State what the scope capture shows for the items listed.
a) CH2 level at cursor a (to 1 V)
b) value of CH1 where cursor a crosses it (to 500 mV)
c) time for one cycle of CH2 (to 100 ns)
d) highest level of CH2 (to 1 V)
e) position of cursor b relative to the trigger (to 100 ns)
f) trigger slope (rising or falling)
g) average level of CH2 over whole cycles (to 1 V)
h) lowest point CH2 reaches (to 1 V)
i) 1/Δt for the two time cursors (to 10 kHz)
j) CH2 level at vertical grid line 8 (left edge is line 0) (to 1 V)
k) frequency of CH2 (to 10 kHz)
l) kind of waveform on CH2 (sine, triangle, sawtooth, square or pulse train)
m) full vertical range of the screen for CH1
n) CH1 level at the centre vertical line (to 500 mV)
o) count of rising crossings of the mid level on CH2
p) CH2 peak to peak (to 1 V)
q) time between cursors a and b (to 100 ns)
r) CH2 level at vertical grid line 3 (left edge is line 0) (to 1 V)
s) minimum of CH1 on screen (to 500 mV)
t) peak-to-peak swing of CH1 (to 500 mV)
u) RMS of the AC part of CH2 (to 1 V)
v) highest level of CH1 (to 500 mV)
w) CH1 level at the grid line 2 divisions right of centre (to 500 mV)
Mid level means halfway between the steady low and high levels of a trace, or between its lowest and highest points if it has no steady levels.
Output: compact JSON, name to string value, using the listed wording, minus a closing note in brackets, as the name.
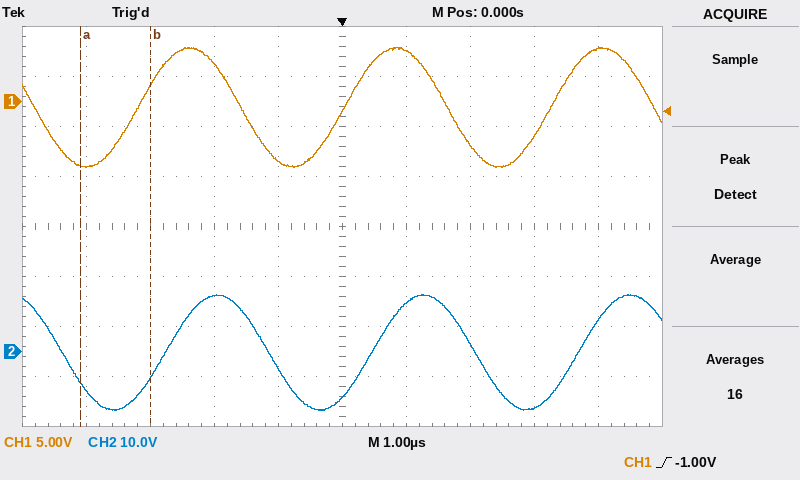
{"CH2 level at cursor a": "-6 V", "value of CH1 where cursor a crosses it": "-6.5 V", "time for one cycle of CH2": "3.2 µs", "highest level of CH2": "11 V", "position of cursor b relative to the trigger": "-3.0 µs", "trigger slope": "rising", "average level of CH2 over whole cycles": "0 V", "lowest point CH2 reaches": "-12 V", "1/Δt for the two time cursors": "910 kHz", "CH2 level at vertical grid line 8 (left edge is line 0)": "-11 V", "frequency of CH2": "310 kHz", "kind of waveform on CH2": "sine", "full vertical range of the screen for CH1": "40 V", "CH1 level at the centre vertical line": "-1.0 V", "count of rising crossings of the mid level on CH2": "3", "CH2 peak to peak": "23 V", "time between cursors a and b": "1.1 µs", "CH2 level at vertical grid line 3 (left edge is line 0)": "11 V", "minimum of CH1 on screen": "-6.5 V", "peak-to-peak swing of CH1": "12.0 V", "RMS of the AC part of CH2": "8 V", "highest level of CH1": "5.5 V", "CH1 level at the grid line 2 divisions right of centre": "-4.5 V"}
